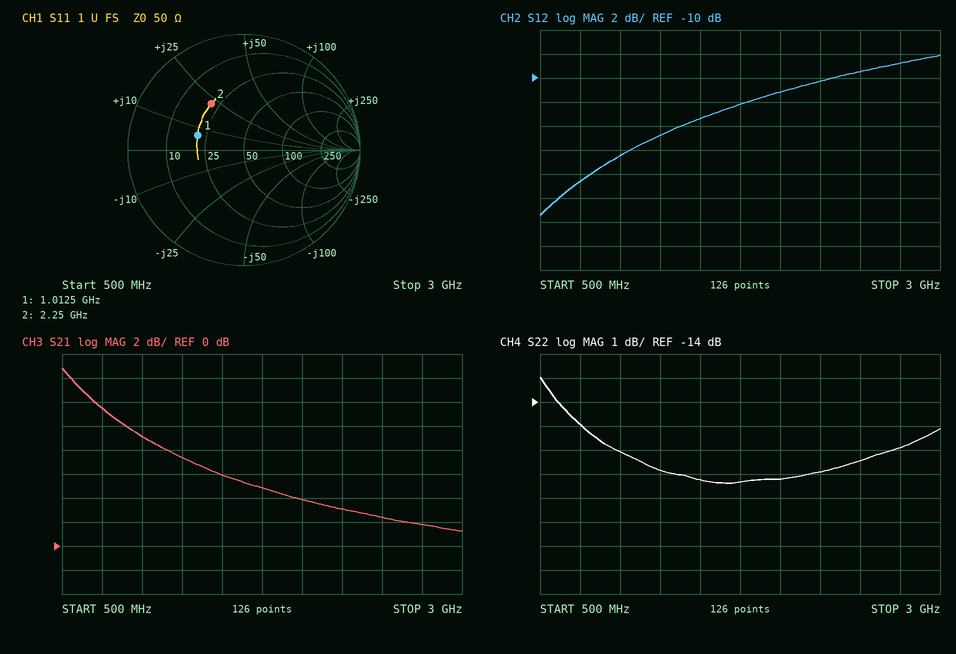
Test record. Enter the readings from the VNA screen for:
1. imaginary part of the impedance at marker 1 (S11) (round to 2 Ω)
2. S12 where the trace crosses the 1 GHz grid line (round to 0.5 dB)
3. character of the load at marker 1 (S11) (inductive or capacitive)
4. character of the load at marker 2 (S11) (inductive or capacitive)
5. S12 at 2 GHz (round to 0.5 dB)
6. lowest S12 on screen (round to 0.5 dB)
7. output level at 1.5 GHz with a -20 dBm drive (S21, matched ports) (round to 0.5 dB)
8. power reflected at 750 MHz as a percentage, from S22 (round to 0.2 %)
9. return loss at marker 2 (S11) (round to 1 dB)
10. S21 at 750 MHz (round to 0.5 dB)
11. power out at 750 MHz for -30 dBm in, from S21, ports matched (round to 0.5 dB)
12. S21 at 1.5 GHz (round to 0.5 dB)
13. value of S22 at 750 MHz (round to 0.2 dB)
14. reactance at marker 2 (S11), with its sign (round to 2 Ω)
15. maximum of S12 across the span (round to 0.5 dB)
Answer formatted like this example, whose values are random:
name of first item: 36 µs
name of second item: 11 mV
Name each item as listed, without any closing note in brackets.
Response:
imaginary part of the impedance at marker 1 (S11): +6 Ω
S12 where the trace crosses the 1 GHz grid line: -16.5 dB
character of the load at marker 1 (S11): inductive
character of the load at marker 2 (S11): inductive
S12 at 2 GHz: -11.0 dB
lowest S12 on screen: -21.5 dB
output level at 1.5 GHz with a -20 dBm drive (S21, matched ports): -14.0 dBm
power reflected at 750 MHz as a percentage, from S22: 3.2 %
return loss at marker 2 (S11): 6 dB
S21 at 750 MHz: 11.5 dB
power out at 750 MHz for -30 dBm in, from S21, ports matched: -18.5 dBm
S21 at 1.5 GHz: 6.0 dB
value of S22 at 750 MHz: -15.0 dB
reactance at marker 2 (S11), with its sign: +22 Ω
maximum of S12 across the span: -8.0 dB
